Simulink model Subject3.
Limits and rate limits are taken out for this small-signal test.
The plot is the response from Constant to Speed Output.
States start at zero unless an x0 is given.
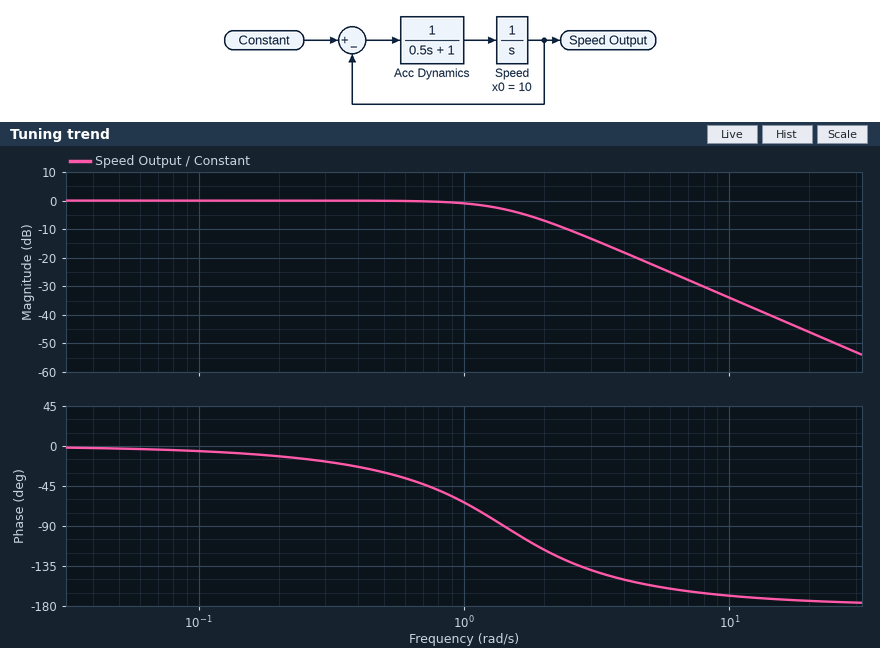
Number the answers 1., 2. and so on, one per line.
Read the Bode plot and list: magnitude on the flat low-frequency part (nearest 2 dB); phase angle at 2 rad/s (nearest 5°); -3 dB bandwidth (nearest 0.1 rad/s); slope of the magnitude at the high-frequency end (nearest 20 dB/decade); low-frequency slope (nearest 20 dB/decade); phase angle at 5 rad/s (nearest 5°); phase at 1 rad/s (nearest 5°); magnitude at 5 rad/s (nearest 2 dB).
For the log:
1. 0 dB
2. -115°
3. 1.4 rad/s
4. -40 dB/decade
5. 0 dB/decade
6. -155°
7. -65°
8. -22 dB
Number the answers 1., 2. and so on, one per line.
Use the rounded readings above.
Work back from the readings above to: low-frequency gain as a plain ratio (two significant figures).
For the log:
1. 1.0
